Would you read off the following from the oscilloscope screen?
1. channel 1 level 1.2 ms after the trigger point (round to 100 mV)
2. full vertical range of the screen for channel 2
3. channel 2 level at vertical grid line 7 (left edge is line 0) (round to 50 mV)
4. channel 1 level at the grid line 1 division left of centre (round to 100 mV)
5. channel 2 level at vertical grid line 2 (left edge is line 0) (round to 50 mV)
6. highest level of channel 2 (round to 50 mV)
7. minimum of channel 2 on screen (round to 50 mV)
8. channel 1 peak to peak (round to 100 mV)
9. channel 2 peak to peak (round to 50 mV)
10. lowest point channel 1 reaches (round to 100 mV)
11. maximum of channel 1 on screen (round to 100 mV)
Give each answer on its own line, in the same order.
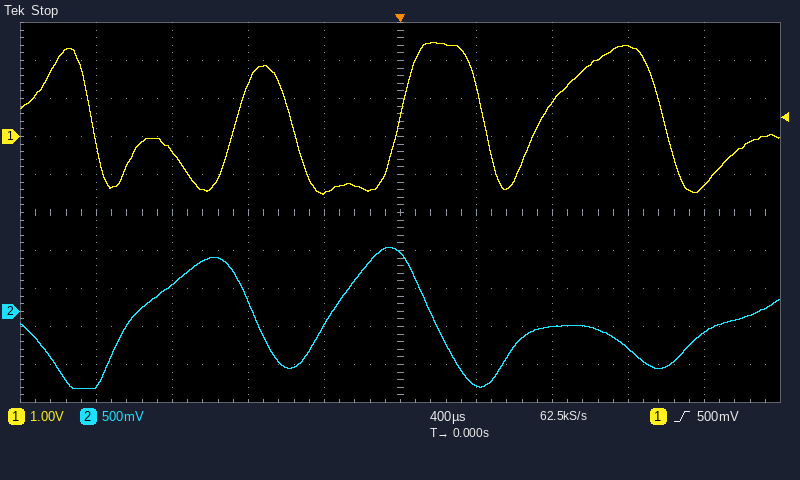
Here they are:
2.4 V
5 V
-200 mV
-1.5 V
350 mV
850 mV
-1.00 V
4.0 V
1.85 V
-1.5 V
2.5 V
